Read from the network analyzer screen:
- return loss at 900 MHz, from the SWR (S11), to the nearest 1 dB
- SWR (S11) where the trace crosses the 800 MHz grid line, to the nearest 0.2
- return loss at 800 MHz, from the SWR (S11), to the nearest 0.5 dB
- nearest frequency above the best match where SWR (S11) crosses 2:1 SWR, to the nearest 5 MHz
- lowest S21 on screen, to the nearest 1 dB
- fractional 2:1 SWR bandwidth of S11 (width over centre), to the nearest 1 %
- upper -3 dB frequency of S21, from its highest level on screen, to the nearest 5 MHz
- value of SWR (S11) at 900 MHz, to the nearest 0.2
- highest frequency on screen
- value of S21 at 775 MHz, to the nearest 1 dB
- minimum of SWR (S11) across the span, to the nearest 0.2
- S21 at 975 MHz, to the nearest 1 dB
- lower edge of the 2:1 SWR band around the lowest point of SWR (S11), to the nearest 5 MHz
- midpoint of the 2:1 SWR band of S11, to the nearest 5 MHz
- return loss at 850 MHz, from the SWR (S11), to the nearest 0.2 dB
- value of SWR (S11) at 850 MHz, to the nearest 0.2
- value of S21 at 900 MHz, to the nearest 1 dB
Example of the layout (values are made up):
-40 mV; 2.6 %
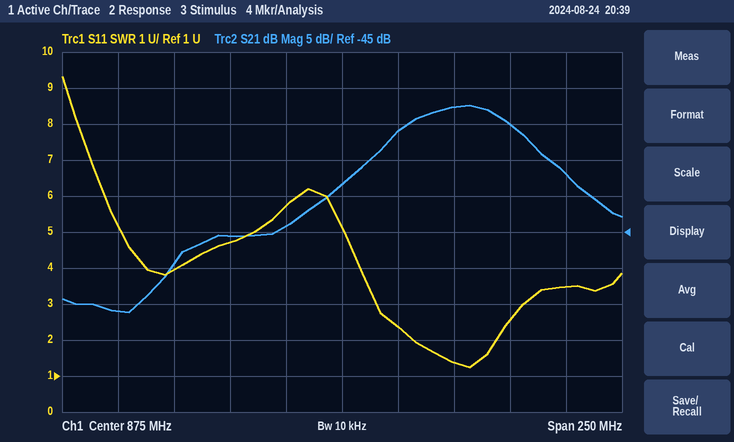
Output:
8 dB; 4.0; 4.5 dB; 945 MHz; -56 dB; 4 %; 950 MHz; 2.4; 1 GHz; -56 dB; 1.2; -37 dB; 905 MHz; 925 MHz; 3.0 dB; 5.8; -31 dB
